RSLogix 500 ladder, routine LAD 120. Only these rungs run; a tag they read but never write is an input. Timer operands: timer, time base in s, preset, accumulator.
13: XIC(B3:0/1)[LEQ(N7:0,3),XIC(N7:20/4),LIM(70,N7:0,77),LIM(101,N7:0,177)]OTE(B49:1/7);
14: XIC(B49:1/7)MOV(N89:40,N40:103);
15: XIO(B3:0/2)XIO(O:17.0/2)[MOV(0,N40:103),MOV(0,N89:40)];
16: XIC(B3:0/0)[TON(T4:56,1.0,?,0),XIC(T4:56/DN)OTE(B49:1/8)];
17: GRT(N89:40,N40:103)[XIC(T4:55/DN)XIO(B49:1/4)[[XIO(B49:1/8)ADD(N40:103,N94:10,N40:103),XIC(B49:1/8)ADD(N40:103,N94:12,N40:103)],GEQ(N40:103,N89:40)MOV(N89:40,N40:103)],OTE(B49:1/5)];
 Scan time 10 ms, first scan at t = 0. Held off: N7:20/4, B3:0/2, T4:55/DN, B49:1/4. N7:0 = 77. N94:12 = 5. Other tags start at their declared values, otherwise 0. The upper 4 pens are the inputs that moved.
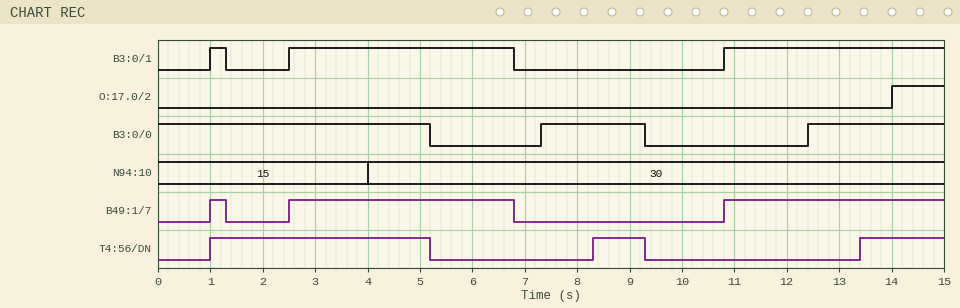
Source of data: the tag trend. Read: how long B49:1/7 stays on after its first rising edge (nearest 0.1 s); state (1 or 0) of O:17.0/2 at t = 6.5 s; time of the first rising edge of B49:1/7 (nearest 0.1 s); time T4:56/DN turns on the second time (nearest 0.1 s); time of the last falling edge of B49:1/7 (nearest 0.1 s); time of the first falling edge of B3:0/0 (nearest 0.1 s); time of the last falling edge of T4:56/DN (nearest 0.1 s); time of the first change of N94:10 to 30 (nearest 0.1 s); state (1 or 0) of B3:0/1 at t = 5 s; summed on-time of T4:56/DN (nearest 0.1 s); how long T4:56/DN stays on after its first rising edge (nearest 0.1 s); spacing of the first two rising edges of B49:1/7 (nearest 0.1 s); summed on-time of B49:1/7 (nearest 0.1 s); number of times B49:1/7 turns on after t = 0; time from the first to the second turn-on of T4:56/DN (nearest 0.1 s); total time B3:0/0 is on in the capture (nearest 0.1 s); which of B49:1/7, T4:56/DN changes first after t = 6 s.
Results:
0.3 s
0
1.0 s
8.3 s
6.8 s
5.2 s
9.3 s
4.0 s
1
6.8 s
4.2 s
1.5 s
8.8 s
3
7.3 s
9.8 s
B49:1/7
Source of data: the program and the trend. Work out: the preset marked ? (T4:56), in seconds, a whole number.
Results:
1 s
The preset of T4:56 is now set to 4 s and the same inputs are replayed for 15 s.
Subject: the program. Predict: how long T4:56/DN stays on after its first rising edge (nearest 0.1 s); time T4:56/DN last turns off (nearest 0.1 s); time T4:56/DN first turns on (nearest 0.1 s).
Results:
1.2 s
5.2 s
4.0 s
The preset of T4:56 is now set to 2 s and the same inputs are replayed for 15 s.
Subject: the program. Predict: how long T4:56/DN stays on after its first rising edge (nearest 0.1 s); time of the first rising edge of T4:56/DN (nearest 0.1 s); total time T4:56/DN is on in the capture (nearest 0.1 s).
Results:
3.2 s
2.0 s
3.8 s
